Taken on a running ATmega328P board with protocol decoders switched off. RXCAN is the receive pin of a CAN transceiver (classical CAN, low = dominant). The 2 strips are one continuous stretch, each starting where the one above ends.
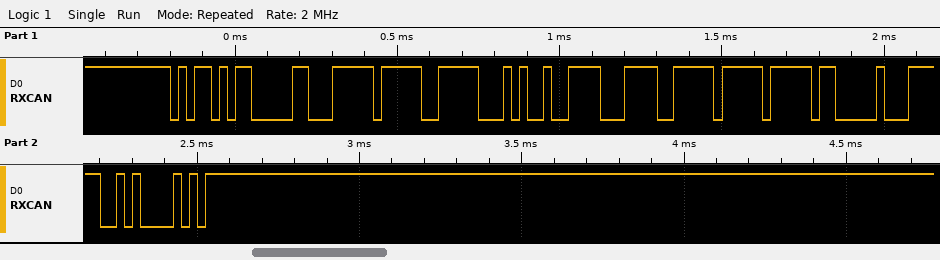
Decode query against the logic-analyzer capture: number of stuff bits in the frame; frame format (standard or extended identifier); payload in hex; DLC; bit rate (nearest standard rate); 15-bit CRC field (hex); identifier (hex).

9
standard
FF DF 29 3C 79 FF FF 00
8
40 kbit/s
0x7D42
0x5AC
